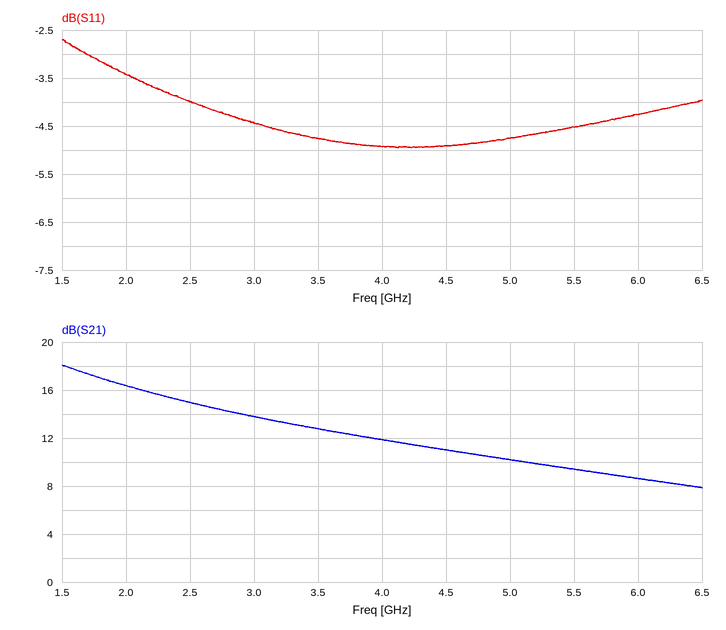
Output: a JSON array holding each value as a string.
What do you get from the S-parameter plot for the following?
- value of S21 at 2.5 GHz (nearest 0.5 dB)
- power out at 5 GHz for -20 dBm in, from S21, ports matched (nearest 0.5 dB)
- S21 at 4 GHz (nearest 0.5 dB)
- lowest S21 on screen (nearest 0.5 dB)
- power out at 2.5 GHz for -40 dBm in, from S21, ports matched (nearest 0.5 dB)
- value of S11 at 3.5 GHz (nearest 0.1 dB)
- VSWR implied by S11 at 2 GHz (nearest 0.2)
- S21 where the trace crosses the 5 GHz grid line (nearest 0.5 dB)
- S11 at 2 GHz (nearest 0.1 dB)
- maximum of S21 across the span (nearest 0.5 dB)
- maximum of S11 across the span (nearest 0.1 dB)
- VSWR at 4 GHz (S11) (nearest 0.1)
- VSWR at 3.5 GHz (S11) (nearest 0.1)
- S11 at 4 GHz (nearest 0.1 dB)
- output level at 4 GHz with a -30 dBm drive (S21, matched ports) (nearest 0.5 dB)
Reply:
["15.0 dB", "-10.0 dBm", "12.0 dB", "8.0 dB", "-25.0 dBm", "-4.8 dB", "5.2", "10.0 dB", "-3.4 dB", "18.0 dB", "-2.7 dB", "3.6", "3.7", "-4.9 dB", "-18.0 dBm"]
